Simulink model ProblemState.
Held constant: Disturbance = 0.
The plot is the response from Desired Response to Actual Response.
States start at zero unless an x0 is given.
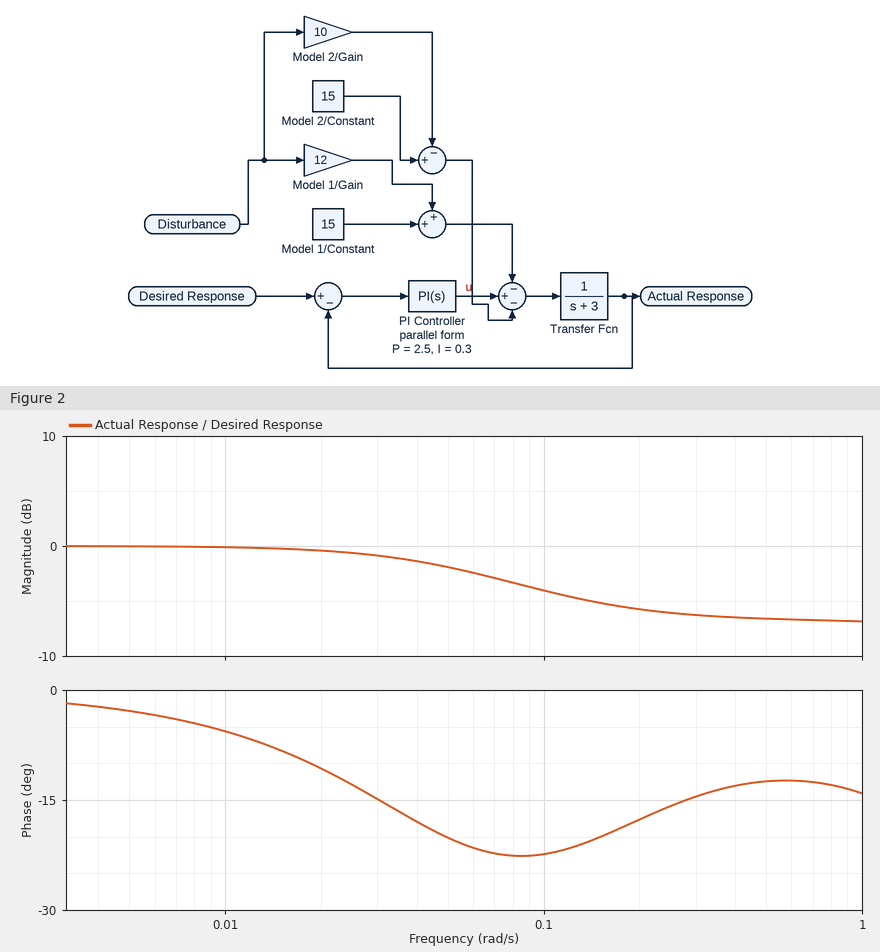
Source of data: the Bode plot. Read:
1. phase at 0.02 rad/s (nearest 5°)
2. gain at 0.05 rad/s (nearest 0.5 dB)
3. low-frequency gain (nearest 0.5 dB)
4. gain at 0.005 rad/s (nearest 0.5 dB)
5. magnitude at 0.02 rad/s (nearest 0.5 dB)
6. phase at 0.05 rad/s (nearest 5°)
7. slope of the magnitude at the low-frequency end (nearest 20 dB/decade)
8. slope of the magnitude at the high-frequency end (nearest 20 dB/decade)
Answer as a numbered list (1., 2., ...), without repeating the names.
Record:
1. -10°
2. -2.0 dB
3. 0.0 dB
4. 0.0 dB
5. -0.5 dB
6. -20°
7. 0 dB/decade
8. 0 dB/decade
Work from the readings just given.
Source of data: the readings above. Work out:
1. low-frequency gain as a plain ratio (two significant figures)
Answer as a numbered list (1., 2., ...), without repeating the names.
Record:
1. 1.0
